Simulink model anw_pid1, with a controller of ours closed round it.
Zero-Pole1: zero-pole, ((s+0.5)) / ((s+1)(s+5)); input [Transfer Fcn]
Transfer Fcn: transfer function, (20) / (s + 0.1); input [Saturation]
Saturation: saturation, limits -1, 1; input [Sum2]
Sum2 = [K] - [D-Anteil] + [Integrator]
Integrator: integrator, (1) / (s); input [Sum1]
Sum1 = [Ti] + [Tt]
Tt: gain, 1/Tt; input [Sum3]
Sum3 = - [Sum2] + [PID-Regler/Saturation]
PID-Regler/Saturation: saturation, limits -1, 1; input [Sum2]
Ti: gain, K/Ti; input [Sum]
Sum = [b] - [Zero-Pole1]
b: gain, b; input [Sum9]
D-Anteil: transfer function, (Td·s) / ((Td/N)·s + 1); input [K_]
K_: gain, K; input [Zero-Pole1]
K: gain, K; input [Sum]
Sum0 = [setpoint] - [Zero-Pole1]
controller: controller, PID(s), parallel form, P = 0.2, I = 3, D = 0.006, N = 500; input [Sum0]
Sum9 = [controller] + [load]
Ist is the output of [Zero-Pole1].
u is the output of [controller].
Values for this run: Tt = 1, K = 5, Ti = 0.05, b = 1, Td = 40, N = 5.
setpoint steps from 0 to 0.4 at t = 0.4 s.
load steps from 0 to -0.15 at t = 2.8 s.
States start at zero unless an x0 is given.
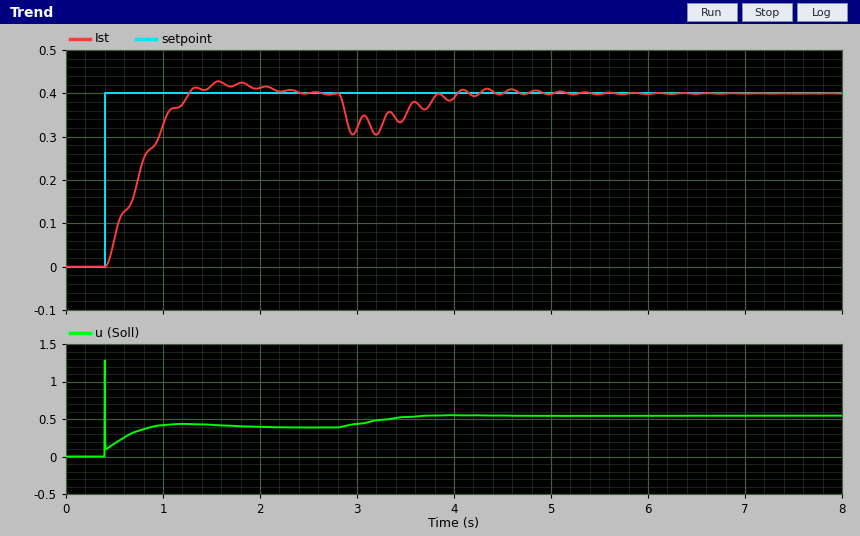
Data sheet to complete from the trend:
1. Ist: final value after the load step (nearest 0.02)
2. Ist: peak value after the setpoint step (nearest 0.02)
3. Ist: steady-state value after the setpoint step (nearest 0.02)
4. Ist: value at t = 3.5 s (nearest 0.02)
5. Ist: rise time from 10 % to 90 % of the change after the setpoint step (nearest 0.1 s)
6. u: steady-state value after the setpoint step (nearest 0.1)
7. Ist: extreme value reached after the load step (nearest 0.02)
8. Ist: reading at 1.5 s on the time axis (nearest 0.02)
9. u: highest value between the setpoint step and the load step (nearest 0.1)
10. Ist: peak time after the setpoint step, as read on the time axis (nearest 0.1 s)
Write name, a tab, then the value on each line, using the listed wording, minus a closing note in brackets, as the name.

Ist: final value after the load step	0.40
Ist: peak value after the setpoint step	0.42
Ist: steady-state value after the setpoint step	0.40
Ist: value at t = 3.5 s	0.34
Ist: rise time from 10 % to 90 % of the change after the setpoint step	0.6 s
u: steady-state value after the setpoint step	0.4
Ist: extreme value reached after the load step	0.30
Ist: reading at 1.5 s on the time axis	0.42
u: highest value between the setpoint step and the load step	1.3
Ist: peak time after the setpoint step, as read on the time axis	1.6 s
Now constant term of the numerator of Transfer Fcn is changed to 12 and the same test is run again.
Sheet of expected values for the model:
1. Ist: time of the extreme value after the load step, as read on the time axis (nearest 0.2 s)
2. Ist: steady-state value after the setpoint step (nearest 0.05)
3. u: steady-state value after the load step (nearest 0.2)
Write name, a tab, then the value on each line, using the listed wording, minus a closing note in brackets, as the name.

Ist: time of the extreme value after the load step, as read on the time axis	3.0 s
Ist: steady-state value after the setpoint step	0.40
u: steady-state value after the load step	0.6
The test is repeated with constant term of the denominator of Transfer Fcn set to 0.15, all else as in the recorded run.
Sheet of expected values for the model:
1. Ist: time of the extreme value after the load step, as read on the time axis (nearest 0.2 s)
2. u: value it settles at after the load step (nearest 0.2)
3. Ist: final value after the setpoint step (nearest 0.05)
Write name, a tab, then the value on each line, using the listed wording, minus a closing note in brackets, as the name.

Ist: time of the extreme value after the load step, as read on the time axis	3.2 s
u: value it settles at after the load step	0.6
Ist: final value after the setpoint step	0.40
